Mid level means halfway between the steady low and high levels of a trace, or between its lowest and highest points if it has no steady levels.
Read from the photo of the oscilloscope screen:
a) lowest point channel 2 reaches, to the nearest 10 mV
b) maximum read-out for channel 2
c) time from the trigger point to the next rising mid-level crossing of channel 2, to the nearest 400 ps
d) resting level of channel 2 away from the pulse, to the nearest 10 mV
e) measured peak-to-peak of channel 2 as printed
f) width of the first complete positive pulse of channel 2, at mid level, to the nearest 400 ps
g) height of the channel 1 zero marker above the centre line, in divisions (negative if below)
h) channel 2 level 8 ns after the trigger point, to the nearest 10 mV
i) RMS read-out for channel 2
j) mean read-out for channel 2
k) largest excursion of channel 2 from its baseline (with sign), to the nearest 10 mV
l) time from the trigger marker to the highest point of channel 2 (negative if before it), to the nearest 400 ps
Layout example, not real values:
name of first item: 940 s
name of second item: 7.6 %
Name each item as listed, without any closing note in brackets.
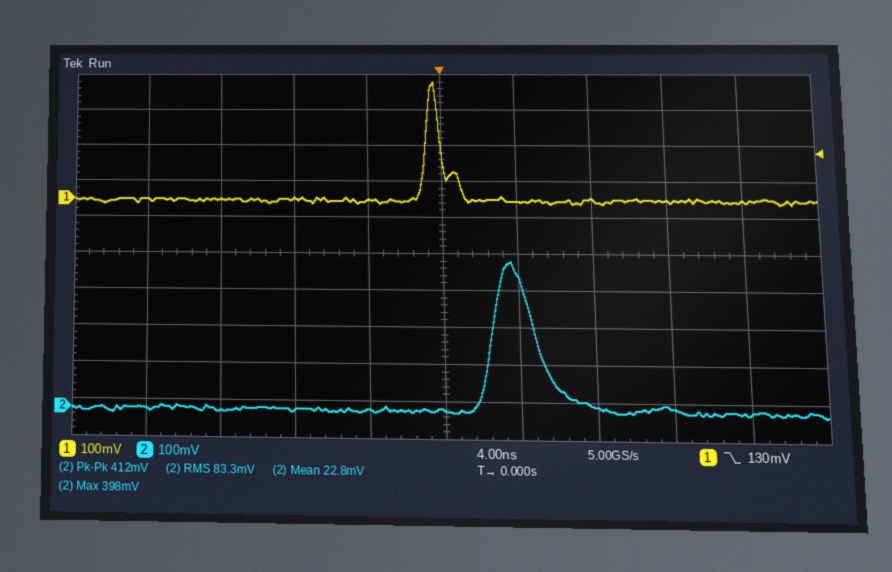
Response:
lowest point channel 2 reaches, to the nearest 10 mV: -10 mV
maximum read-out for channel 2: 398 mV
time from the trigger point to the next rising mid-level crossing of channel 2, to the nearest 400 ps: 2.4 ns
resting level of channel 2 away from the pulse, to the nearest 10 mV: 0 mV
measured peak-to-peak of channel 2 as printed: 412 mV
width of the first complete positive pulse of channel 2, at mid level, to the nearest 400 ps: 2.4 ns
height of the channel 1 zero marker above the centre line, in divisions: +1.5 div
channel 2 level 8 ns after the trigger point, to the nearest 10 mV: 10 mV
RMS read-out for channel 2: 83.3 mV
mean read-out for channel 2: 22.8 mV
largest excursion of channel 2 from its baseline (with sign), to the nearest 10 mV: +400 mV
time from the trigger marker to the highest point of channel 2 (negative if before it), to the nearest 400 ps: +3.6 ns
